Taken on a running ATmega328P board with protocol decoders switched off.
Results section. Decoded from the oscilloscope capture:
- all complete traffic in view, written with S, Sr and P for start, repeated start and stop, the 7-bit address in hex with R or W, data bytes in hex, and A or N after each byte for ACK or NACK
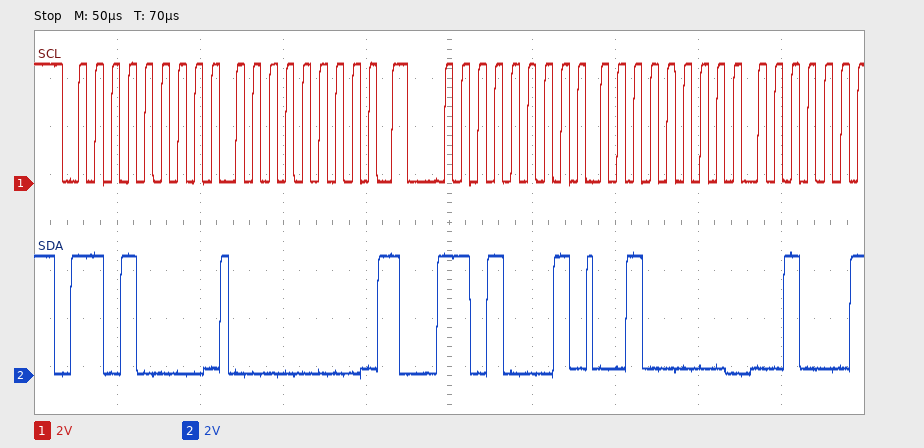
S 68W A 00 A Sr 68R A 20 A
